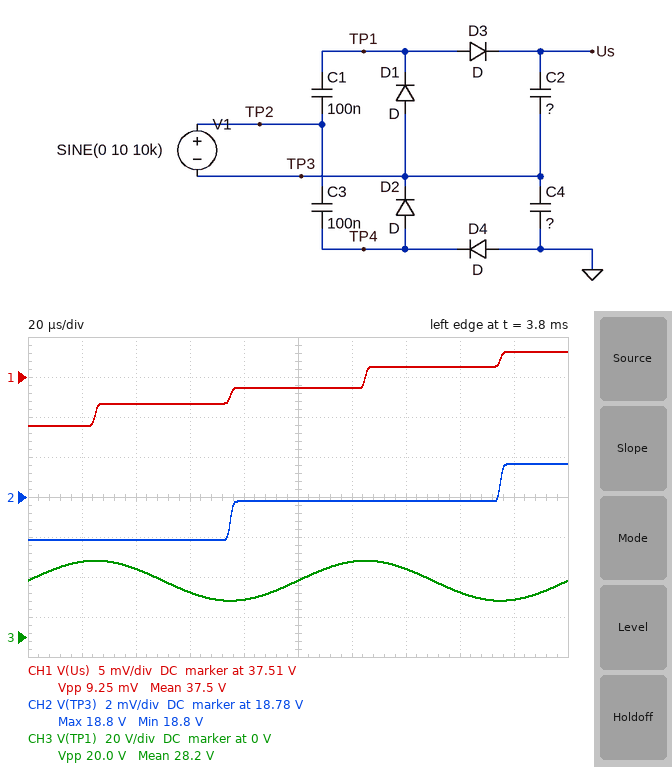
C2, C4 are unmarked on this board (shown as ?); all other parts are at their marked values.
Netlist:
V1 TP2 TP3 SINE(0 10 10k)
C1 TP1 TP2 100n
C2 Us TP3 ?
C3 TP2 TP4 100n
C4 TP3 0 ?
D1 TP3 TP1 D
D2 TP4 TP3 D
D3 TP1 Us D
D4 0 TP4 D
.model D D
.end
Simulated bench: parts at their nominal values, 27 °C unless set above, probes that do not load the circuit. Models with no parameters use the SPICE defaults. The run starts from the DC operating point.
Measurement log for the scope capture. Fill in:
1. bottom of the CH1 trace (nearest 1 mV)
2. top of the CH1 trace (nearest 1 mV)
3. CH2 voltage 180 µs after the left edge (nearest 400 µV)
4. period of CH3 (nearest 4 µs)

37.499 V
37.508 V
18.7776 V
100 µs
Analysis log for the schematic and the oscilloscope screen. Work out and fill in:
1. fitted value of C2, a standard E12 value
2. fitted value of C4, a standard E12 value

330 nF
180 nF
